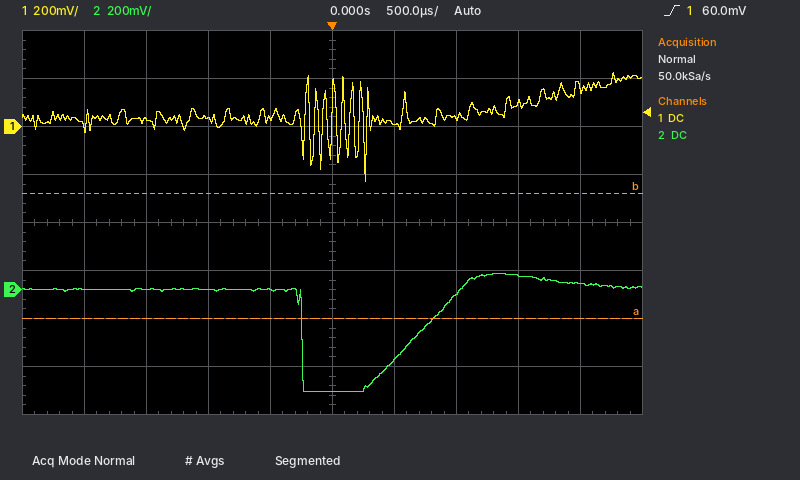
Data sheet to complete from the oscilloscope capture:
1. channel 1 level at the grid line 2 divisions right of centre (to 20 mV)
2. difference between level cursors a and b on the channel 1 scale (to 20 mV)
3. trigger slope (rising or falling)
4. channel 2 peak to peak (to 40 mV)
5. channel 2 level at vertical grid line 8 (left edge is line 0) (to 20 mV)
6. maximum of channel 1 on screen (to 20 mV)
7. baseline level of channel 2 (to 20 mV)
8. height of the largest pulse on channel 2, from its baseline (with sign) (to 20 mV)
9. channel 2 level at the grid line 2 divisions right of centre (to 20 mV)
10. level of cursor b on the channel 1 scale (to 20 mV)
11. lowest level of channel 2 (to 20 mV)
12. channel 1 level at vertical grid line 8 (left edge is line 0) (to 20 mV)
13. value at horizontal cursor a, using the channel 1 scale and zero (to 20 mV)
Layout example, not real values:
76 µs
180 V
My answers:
40 mV
520 mV
rising
480 mV
60 mV
220 mV
0 mV
-420 mV
-20 mV
-280 mV
-420 mV
100 mV
-800 mV
